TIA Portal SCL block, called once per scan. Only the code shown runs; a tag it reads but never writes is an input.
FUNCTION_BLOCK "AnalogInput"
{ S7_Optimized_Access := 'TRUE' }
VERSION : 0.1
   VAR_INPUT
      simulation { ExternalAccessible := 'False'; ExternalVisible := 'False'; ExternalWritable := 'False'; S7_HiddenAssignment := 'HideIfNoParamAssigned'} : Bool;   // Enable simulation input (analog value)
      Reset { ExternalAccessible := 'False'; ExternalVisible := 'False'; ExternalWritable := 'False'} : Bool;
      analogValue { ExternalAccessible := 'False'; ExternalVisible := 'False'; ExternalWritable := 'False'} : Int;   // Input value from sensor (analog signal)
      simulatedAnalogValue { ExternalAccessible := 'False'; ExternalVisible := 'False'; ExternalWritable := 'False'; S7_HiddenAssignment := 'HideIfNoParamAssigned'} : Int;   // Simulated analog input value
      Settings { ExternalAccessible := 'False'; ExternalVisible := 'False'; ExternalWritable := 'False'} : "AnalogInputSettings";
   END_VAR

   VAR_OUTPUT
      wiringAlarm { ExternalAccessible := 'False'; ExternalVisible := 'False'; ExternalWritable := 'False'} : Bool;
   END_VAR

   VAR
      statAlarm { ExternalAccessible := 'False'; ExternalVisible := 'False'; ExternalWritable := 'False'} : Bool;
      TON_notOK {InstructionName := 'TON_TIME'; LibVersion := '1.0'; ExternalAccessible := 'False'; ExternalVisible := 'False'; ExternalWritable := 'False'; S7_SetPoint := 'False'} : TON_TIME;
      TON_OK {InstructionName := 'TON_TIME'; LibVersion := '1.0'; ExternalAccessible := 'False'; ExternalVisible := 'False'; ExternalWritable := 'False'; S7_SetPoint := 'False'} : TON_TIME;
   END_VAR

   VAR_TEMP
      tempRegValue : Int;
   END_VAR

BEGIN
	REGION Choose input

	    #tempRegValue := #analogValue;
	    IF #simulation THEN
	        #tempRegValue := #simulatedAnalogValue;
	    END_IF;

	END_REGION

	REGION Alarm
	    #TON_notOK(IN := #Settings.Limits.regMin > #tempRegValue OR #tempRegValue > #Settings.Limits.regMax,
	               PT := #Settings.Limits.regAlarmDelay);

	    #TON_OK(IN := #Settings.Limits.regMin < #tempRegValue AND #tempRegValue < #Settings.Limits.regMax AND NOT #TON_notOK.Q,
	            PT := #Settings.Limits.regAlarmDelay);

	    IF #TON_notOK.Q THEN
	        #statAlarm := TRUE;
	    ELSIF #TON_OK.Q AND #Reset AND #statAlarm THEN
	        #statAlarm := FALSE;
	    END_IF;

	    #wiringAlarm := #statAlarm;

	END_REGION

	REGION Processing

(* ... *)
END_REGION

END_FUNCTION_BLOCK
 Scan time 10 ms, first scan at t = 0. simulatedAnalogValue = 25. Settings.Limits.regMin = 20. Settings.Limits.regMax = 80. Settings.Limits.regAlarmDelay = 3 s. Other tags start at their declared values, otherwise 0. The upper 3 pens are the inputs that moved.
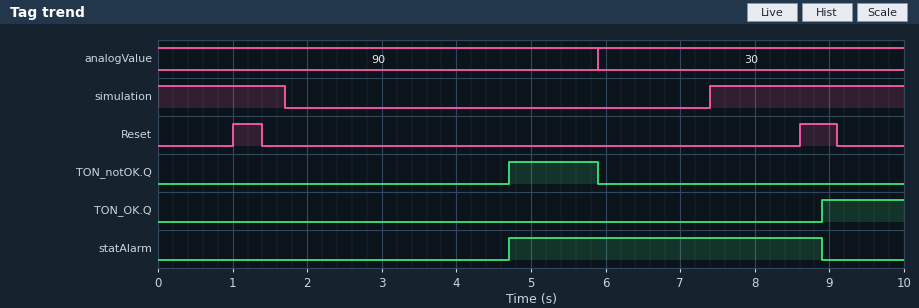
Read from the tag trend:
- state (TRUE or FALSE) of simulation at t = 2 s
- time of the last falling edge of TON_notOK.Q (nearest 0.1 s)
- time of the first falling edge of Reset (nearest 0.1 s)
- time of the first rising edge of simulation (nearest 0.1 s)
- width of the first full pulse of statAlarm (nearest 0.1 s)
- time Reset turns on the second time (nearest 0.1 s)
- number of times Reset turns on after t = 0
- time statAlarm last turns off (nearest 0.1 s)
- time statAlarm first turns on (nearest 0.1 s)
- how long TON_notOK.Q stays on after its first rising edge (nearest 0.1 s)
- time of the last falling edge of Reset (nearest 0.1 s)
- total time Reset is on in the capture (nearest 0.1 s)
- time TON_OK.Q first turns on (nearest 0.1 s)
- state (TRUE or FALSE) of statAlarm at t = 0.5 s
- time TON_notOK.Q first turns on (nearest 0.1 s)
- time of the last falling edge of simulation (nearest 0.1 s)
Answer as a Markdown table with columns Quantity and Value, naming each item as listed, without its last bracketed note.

| Quantity | Value |
|---|---|
| state (TRUE or FALSE) of simulation at t = 2 s | FALSE |
| time of the last falling edge of TON_notOK.Q | 5.9 s |
| time of the first falling edge of Reset | 1.4 s |
| time of the first rising edge of simulation | 7.4 s |
| width of the first full pulse of statAlarm | 4.2 s |
| time Reset turns on the second time | 8.6 s |
| number of times Reset turns on after t = 0 | 2 |
| time statAlarm last turns off | 8.9 s |
| time statAlarm first turns on | 4.7 s |
| how long TON_notOK.Q stays on after its first rising edge | 1.2 s |
| time of the last falling edge of Reset | 9.1 s |
| total time Reset is on in the capture | 0.9 s |
| time TON_OK.Q first turns on | 8.9 s |
| state (TRUE or FALSE) of statAlarm at t = 0.5 s | FALSE |
| time TON_notOK.Q first turns on | 4.7 s |
| time of the last falling edge of simulation | 1.7 s |
